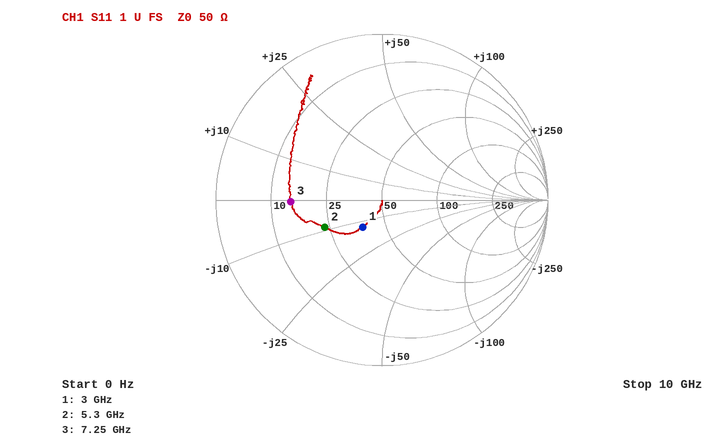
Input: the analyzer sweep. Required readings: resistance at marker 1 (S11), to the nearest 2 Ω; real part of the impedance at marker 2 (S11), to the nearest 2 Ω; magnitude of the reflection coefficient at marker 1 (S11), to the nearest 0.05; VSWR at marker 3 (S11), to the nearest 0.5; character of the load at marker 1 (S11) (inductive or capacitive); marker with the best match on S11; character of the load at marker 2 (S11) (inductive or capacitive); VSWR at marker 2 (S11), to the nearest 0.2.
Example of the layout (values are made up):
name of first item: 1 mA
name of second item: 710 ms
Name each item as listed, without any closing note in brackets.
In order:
resistance at marker 1 (S11), to the nearest 2 Ω: 38 Ω
real part of the impedance at marker 2 (S11), to the nearest 2 Ω: 24 Ω
magnitude of the reflection coefficient at marker 1 (S11), to the nearest 0.05: 0.20
VSWR at marker 3 (S11), to the nearest 0.5: 3.5
character of the load at marker 1 (S11): capacitive
marker with the best match on S11: marker 1
character of the load at marker 2 (S11): capacitive
VSWR at marker 2 (S11), to the nearest 0.2: 2.2
